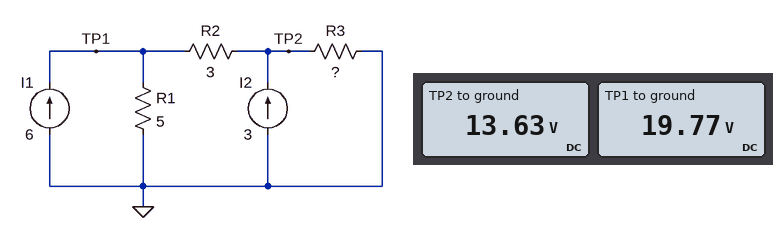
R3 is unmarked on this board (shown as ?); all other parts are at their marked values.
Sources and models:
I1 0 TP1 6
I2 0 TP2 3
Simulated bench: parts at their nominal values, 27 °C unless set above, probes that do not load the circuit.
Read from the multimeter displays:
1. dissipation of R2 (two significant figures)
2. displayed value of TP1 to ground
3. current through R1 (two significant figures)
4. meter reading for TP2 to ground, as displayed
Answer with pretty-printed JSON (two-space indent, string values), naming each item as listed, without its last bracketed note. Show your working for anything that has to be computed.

{
  "dissipation of R2": "(19.77 V - 13.63 V)^2 / 3 Ω = 13 W",
  "displayed value of TP1 to ground": "19.77 V",
  "current through R1": "(19.77 V) / 5 Ω = 4.0 A",
  "meter reading for TP2 to ground, as displayed": "13.63 V"
}
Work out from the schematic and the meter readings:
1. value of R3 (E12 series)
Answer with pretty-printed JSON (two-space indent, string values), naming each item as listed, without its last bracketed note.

{
  "value of R3": "2.7 Ω"
}
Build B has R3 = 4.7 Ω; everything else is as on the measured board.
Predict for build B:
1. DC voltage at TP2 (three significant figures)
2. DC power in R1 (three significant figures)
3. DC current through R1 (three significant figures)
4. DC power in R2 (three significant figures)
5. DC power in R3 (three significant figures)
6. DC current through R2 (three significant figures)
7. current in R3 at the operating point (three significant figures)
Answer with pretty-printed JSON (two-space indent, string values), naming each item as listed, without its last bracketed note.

{
  "DC voltage at TP2": "20.0 V",
  "DC power in R1": "113 W",
  "DC current through R1": "4.75 A",
  "DC power in R2": "4.70 W",
  "DC power in R3": "85.0 W",
  "DC current through R2": "1.25 A",
  "current in R3 at the operating point": "4.25 A"
}
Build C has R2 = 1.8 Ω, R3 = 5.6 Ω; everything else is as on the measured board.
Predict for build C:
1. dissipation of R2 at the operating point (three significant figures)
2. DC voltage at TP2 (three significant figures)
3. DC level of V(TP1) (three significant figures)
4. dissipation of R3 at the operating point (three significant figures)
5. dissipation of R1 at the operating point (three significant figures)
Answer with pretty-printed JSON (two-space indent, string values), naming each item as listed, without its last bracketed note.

{
  "dissipation of R2 at the operating point": "2.04 W",
  "DC voltage at TP2": "22.8 V",
  "DC level of V(TP1)": "24.7 V",
  "dissipation of R3 at the operating point": "92.5 W",
  "dissipation of R1 at the operating point": "122 W"
}
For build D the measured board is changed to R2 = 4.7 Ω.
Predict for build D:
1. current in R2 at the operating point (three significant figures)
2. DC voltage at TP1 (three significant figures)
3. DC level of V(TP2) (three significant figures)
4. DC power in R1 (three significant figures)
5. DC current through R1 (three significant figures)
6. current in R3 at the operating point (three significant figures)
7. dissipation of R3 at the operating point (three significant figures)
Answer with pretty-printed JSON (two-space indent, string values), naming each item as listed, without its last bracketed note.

{
  "current in R2 at the operating point": "1.77 A",
  "DC voltage at TP1": "21.2 V",
  "DC level of V(TP2)": "12.9 V",
  "DC power in R1": "89.6 W",
  "DC current through R1": "4.23 A",
  "current in R3 at the operating point": "4.77 A",
  "dissipation of R3 at the operating point": "61.3 W"
}
